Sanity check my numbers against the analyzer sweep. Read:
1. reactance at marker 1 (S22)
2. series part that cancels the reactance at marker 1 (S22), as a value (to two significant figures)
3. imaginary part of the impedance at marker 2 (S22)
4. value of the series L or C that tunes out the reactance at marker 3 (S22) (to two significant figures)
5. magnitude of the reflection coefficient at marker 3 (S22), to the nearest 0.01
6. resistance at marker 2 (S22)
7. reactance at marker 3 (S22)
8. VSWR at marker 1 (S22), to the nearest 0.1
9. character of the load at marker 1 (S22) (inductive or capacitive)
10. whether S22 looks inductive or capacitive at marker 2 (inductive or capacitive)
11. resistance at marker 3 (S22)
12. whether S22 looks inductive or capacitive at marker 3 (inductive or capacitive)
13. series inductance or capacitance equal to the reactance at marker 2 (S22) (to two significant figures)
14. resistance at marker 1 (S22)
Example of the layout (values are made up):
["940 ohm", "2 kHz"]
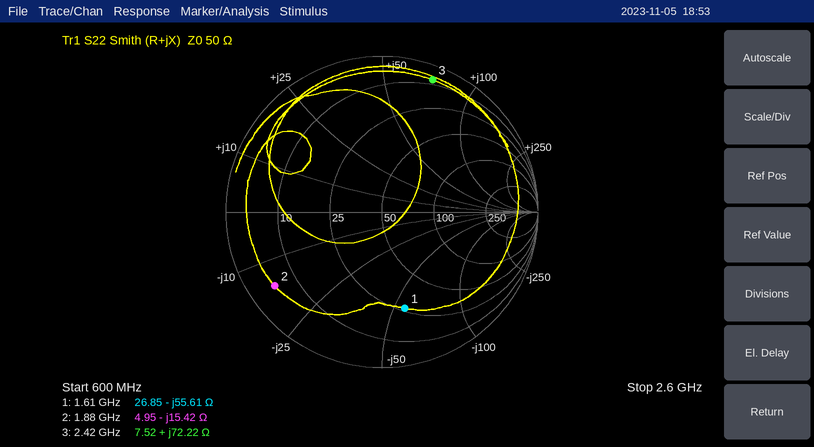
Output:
["-55.61 Ω", "5.5 nH", "-15.42 Ω", "910 fF", "0.91", "4.95 Ω", "+72.22 Ω", "4.5", "capacitive", "capacitive", "7.52 Ω", "inductive", "5.5 pF", "26.85 Ω"]
